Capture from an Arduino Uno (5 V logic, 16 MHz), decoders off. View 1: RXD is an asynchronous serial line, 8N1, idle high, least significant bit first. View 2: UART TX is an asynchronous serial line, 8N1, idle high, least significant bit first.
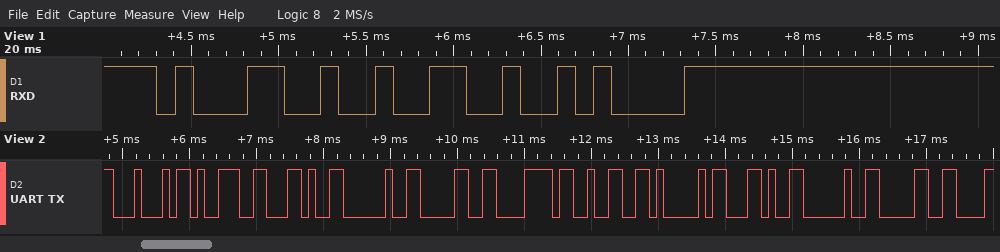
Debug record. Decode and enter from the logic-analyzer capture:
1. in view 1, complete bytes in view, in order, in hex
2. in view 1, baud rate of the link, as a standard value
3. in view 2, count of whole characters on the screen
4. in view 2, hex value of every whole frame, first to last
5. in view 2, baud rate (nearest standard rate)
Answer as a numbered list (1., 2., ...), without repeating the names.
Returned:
1. 31 32 0A
2. 9600 baud
3. 11
4. 0x44 0x39 0x2C 0x20 0x30 0x78 0x32 0x41 0x2C 0x20 0x30
5. 9600 baud
